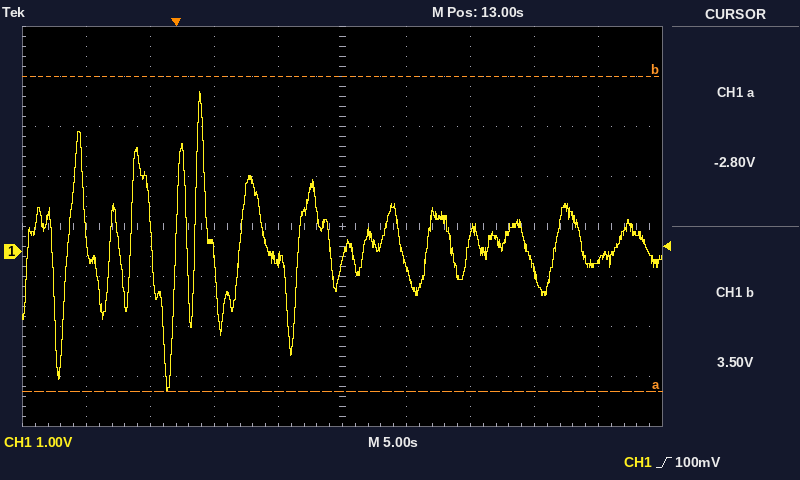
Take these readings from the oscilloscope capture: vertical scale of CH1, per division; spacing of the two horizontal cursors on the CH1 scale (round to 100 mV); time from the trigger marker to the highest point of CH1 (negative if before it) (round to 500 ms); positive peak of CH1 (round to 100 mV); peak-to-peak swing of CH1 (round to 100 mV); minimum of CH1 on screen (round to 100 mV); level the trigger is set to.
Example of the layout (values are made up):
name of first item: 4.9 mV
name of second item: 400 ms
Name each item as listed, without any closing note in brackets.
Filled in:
vertical scale of CH1, per division: 1 V
spacing of the two horizontal cursors on the CH1 scale: 6.3 V
time from the trigger marker to the highest point of CH1 (negative if before it): +2.0 s
positive peak of CH1: 3.2 V
peak-to-peak swing of CH1: 6.0 V
minimum of CH1 on screen: -2.8 V
level the trigger is set to: 100 mV
